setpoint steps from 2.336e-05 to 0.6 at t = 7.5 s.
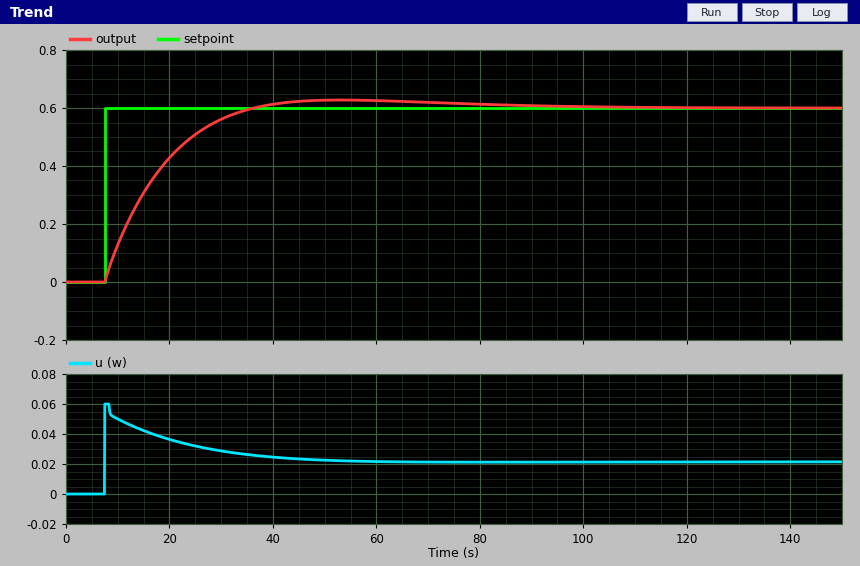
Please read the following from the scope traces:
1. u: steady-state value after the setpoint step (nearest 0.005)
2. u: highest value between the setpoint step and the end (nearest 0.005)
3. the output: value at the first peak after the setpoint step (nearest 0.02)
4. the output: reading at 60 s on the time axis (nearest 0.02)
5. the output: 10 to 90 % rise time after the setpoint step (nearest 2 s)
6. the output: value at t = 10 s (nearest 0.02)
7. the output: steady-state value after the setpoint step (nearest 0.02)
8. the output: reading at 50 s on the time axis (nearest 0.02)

0.020
0.060
0.62
0.62
20 s
0.12
0.60
0.62
